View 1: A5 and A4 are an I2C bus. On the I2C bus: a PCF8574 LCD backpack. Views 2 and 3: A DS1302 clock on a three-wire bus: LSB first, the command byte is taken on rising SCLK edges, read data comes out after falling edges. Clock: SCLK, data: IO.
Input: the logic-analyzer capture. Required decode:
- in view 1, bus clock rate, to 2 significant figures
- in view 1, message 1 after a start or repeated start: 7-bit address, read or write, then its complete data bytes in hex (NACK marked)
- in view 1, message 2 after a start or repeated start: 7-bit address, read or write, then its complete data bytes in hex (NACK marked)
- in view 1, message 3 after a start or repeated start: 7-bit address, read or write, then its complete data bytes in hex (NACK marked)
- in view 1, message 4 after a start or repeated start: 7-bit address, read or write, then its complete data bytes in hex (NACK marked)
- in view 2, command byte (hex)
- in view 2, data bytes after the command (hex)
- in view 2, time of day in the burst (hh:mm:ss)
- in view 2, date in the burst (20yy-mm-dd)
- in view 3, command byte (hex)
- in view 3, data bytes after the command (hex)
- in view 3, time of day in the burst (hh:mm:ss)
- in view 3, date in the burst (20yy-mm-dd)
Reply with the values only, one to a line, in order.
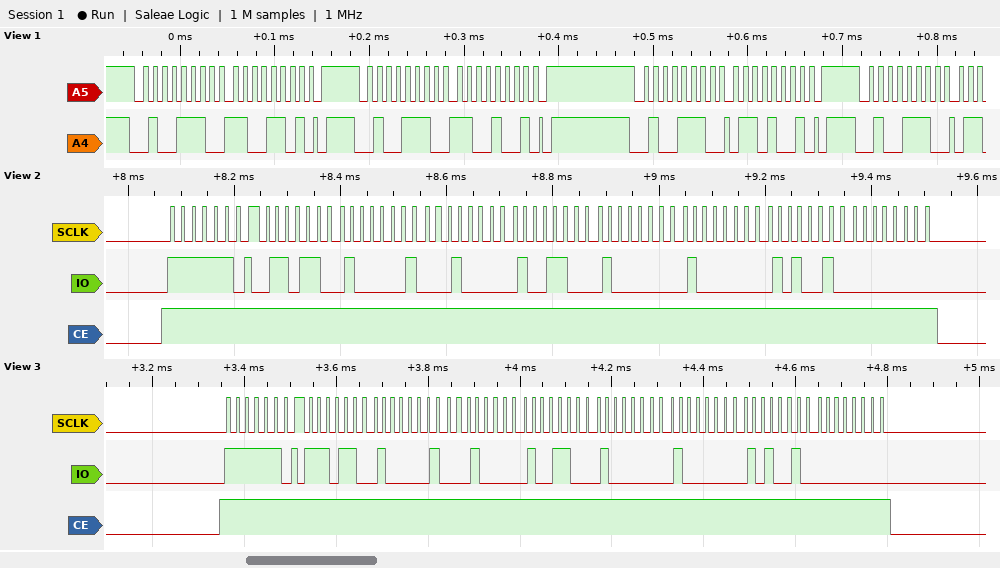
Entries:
100 kHz
0x27 write: CD
0x27 write: C9
0x27 write: 69
0x27 write
0xBF
36 41 04 19 01 01 25 00
04:41:36
2025-01-19
0xBF
37 41 04 19 01 01 25 00
04:41:37
2025-01-19
